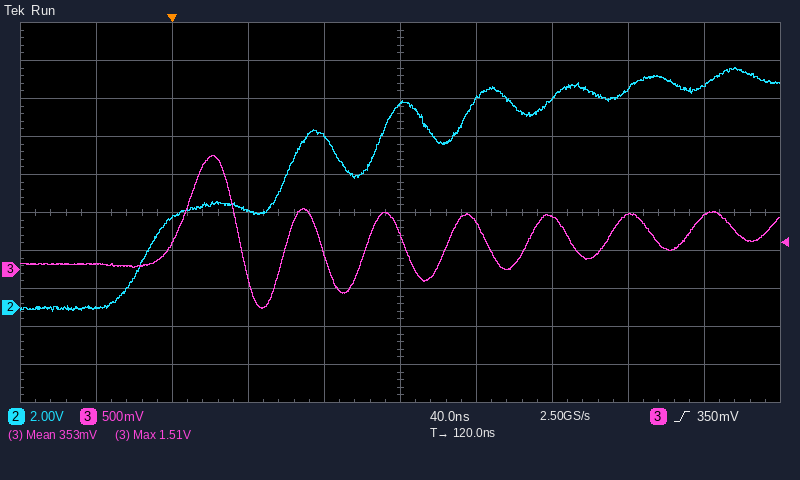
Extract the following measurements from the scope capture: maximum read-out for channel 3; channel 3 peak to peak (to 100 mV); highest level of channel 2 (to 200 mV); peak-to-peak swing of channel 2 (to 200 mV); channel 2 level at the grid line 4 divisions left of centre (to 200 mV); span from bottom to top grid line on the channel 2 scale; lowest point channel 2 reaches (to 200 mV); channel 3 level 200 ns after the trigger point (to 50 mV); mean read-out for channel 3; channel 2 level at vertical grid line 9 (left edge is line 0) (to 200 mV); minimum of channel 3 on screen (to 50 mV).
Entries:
1.51 V
2.00 V
12.6 V
12.8 V
0.0 V
20 V
-200 mV
700 mV
353 mV
11.6 V
-500 mV
